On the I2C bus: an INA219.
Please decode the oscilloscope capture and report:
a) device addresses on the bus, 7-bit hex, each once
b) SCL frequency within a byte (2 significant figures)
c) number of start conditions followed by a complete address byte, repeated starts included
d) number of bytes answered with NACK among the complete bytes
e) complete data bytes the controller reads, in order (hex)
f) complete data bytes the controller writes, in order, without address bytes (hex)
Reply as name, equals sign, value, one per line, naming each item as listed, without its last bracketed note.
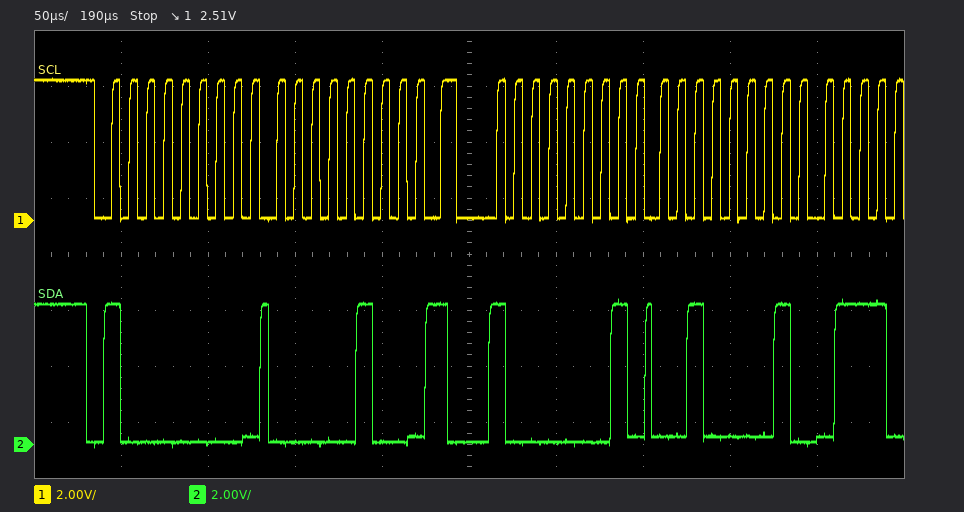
device addresses on the bus, 7-bit hex, each once = 0x40
SCL frequency within a byte = 100 kHz
number of start conditions followed by a complete address byte, repeated starts included = 2
number of bytes answered with NACK among the complete bytes = 0
complete data bytes the controller reads, in order = 21
complete data bytes the controller writes, in order, without address bytes = 04
